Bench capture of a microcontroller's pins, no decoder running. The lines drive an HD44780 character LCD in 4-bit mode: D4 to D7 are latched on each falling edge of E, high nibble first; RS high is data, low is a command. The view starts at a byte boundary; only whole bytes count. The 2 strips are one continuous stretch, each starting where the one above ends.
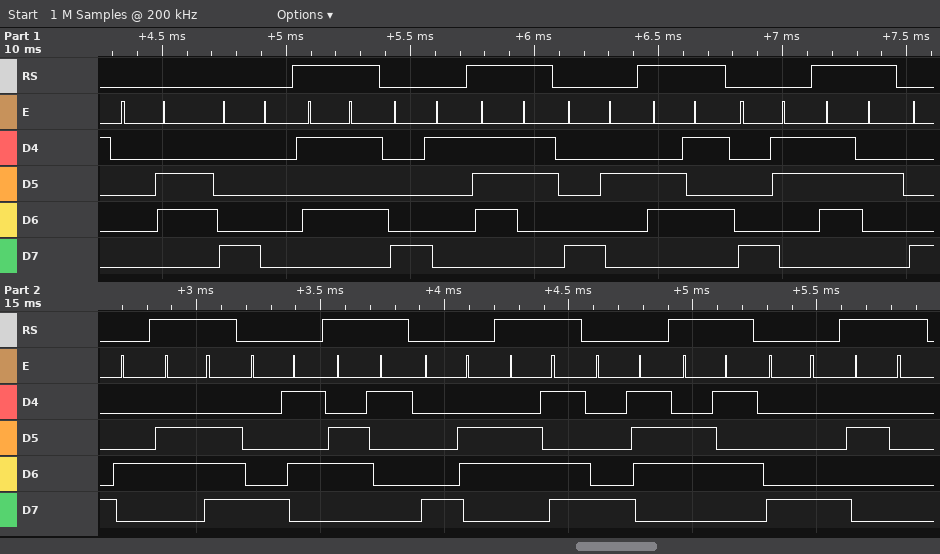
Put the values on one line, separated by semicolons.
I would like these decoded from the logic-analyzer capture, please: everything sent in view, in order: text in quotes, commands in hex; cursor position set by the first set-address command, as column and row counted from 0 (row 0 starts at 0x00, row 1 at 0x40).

0x06 0x80 "U" 0x81 "s" 0x82 "e" 0x83 "r" 0x84 "n" 0x85 "a" 0x86 "m" 0x87 "e" 0x88 " "; column 0, row 0
